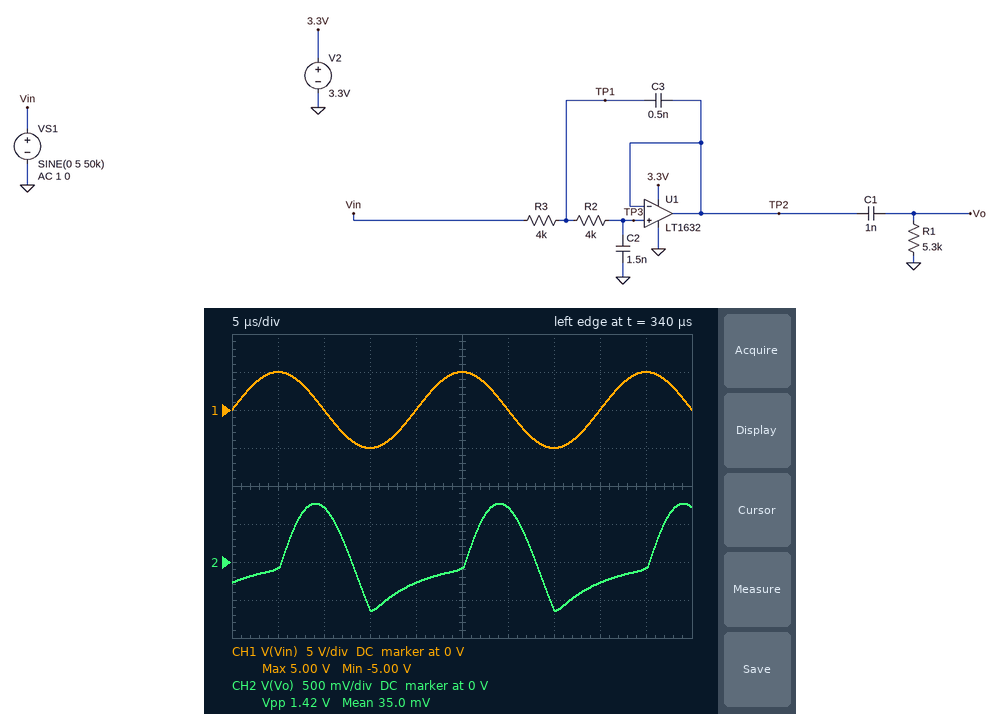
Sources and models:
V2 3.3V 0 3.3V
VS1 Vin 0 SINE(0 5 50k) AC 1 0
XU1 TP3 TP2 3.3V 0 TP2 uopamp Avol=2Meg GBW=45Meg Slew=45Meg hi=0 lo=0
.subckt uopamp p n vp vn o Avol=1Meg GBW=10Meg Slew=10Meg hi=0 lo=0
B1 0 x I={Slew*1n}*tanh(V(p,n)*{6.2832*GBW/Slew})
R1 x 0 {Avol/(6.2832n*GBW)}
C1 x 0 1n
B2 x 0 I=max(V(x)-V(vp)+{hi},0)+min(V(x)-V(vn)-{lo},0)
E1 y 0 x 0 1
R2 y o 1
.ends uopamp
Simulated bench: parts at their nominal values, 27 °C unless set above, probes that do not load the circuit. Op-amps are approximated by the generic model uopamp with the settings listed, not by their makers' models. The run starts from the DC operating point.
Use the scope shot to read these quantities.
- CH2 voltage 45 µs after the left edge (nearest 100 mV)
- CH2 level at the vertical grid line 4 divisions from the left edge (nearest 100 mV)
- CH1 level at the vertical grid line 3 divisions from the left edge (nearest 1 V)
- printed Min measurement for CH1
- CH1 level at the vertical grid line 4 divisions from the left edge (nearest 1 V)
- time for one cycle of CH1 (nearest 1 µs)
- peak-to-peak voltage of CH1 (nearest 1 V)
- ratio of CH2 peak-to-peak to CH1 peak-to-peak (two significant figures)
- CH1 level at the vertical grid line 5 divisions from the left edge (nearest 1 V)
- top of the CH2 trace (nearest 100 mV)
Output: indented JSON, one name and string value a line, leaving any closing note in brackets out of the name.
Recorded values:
{
  "CH2 voltage 45 µs after the left edge": "-100 mV",
  "CH2 level at the vertical grid line 4 divisions from the left edge": "-300 mV",
  "CH1 level at the vertical grid line 3 divisions from the left edge": "-5 V",
  "printed Min measurement for CH1": "-5.00 V",
  "CH1 level at the vertical grid line 4 divisions from the left edge": "0 V",
  "time for one cycle of CH1": "20 µs",
  "peak-to-peak voltage of CH1": "10 V",
  "ratio of CH2 peak-to-peak to CH1 peak-to-peak": "0.14",
  "CH1 level at the vertical grid line 5 divisions from the left edge": "5 V",
  "top of the CH2 trace": "800 mV"
}
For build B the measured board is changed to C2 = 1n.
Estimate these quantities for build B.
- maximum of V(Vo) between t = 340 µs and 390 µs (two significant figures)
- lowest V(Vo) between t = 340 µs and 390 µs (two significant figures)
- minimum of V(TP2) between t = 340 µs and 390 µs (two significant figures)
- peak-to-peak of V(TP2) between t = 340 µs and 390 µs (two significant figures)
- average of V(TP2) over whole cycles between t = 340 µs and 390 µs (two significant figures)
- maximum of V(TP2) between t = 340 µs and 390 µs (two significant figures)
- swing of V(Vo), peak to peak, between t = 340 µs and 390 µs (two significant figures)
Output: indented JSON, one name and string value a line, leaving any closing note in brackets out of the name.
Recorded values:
{
  "maximum of V(Vo) between t = 340 µs and 390 µs": "1.1 V",
  "lowest V(Vo) between t = 340 µs and 390 µs": "-950 mV",
  "minimum of V(TP2) between t = 340 µs and 390 µs": "-45 mV",
  "peak-to-peak of V(TP2) between t = 340 µs and 390 µs": "1.9 V",
  "average of V(TP2) over whole cycles between t = 340 µs and 390 µs": "540 mV",
  "maximum of V(TP2) between t = 340 µs and 390 µs": "1.8 V",
  "swing of V(Vo), peak to peak, between t = 340 µs and 390 µs": "2.1 V"
}
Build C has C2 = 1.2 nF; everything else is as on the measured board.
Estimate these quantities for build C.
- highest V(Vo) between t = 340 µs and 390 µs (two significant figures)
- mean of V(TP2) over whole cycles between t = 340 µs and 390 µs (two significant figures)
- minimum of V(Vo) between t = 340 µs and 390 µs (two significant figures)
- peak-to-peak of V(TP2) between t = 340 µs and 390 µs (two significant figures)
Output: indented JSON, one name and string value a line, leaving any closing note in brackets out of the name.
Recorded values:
{
  "highest V(Vo) between t = 340 µs and 390 µs": "950 mV",
  "mean of V(TP2) over whole cycles between t = 340 µs and 390 µs": "460 mV",
  "minimum of V(Vo) between t = 340 µs and 390 µs": "-800 mV",
  "peak-to-peak of V(TP2) between t = 340 µs and 390 µs": "1.6 V"
}
